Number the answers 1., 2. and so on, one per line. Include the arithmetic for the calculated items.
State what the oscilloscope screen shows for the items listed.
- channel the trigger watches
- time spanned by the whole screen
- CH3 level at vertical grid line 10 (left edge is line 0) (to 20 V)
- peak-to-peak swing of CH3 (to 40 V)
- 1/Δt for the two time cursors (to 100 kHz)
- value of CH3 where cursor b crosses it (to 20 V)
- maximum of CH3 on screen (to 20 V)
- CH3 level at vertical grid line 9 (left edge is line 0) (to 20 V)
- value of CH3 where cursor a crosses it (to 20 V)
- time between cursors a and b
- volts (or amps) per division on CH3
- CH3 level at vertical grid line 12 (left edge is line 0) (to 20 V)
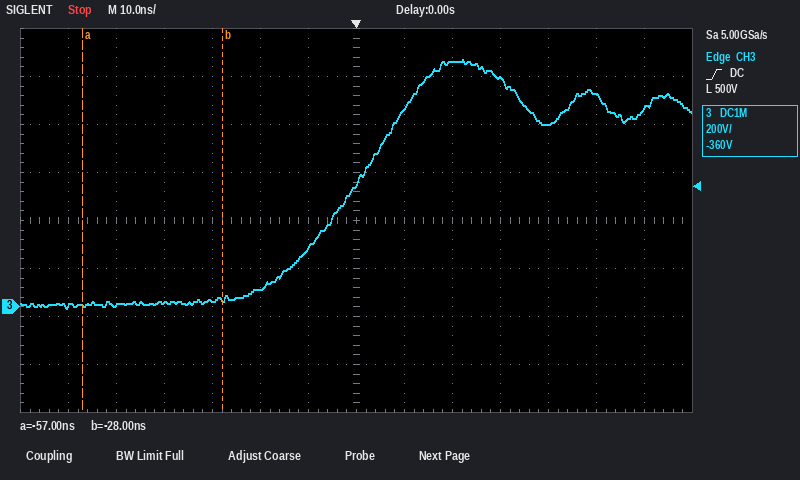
1. CH3
2. 140 ns
3. 960 V
4. 1.04 kV
5. 1 / 29 ns ≈ 34.5 MHz
6. 40 V
7. 1.04 kV
8. 1.02 kV
9. 0 V
10. -28 ns − (-57 ns) = 29 ns
11. 200 V
12. 880 V
